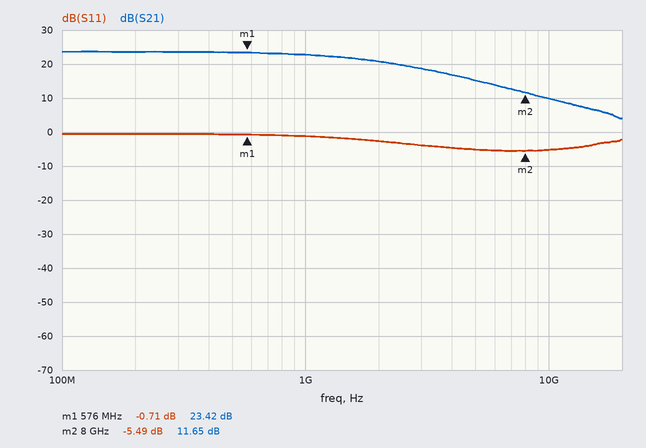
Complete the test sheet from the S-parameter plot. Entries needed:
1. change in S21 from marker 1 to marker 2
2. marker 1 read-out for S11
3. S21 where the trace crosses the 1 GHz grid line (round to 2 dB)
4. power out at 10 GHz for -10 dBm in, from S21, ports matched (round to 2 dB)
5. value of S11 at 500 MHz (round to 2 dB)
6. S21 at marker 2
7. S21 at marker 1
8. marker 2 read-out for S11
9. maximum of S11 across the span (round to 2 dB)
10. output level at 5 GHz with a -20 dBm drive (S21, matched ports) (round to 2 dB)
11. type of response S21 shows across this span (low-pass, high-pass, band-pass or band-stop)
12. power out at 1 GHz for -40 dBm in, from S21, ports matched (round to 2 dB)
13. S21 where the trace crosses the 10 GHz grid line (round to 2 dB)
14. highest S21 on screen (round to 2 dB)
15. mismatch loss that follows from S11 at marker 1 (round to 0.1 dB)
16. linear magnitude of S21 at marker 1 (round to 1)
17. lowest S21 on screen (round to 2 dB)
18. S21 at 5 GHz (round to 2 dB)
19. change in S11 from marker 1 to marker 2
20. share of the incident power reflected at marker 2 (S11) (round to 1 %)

-11.77 dB
-0.71 dB
22 dB
0 dBm
0 dB
11.65 dB
23.42 dB
-5.49 dB
0 dB
-4 dBm
low-pass
-18 dBm
10 dB
24 dB
8.2 dB
15
4 dB
16 dB
-4.78 dB
28 %
